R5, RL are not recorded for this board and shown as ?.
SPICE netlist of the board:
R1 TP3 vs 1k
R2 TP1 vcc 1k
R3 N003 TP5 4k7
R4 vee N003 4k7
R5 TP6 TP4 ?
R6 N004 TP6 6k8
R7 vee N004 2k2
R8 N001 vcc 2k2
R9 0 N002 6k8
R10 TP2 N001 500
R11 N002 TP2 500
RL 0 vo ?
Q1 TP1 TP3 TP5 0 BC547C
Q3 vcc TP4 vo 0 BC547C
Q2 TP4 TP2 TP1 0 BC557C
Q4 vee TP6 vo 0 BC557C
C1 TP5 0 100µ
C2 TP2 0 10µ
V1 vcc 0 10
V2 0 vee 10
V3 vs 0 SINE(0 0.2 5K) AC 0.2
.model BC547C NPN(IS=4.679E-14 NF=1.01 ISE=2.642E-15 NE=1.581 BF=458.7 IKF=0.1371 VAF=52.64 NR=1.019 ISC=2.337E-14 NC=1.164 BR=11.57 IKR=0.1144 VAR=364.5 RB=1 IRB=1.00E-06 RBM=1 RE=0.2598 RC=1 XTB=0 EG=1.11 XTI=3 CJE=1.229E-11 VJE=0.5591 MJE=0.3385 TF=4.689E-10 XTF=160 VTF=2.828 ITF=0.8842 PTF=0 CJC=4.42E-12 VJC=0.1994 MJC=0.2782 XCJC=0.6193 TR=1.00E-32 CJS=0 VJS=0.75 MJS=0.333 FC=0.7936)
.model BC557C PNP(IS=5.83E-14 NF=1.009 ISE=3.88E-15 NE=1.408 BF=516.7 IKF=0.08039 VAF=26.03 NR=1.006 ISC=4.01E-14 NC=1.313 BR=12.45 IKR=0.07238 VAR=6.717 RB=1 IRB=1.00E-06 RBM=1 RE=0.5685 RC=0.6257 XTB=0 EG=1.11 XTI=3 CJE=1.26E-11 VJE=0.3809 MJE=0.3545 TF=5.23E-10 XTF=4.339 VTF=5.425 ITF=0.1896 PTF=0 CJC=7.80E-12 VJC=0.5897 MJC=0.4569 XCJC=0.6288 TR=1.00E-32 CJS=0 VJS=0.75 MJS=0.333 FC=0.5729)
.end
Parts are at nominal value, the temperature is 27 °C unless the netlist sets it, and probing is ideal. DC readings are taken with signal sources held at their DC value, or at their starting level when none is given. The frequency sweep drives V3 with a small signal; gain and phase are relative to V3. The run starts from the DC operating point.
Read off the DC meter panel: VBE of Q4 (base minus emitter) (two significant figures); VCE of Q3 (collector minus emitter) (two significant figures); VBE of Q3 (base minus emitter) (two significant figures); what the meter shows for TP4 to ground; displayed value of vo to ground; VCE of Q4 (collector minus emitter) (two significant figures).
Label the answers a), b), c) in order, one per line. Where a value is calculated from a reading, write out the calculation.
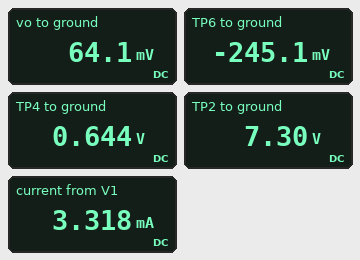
a) -245.1 mV - 64.1 mV = -310 mV
b) 10 V - 64.1 mV = 9.9 V
c) 644 mV - 64.1 mV = 580 mV
d) 0.644 V
e) 64.1 mV
f) -10 V - 64.1 mV = -10 V
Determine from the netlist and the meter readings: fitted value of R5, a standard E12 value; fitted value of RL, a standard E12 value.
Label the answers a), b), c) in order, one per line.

a) 820 Ω
b) 270 Ω
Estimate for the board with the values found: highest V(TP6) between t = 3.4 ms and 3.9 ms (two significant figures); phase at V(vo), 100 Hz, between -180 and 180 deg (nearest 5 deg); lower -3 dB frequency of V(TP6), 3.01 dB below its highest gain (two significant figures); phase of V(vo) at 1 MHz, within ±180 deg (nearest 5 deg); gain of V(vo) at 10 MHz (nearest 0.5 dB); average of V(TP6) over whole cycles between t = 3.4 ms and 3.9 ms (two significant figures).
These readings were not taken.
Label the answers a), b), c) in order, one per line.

a) 6.5 V
b) -150 deg
c) 56 Hz
d) 115 deg
e) 17.5 dB
f) 920 mV
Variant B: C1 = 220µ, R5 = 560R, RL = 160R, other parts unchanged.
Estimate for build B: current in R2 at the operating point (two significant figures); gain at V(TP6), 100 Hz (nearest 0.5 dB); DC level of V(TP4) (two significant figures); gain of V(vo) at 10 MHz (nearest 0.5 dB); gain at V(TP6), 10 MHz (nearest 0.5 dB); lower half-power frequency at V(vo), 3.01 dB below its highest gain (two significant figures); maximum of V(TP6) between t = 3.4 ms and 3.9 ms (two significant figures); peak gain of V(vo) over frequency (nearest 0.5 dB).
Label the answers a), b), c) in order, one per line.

a) 2.1 mA
b) 49.5 dB
c) 370 mV
d) 3.0 dB
e) 11.0 dB
f) 340 kHz
g) 6.9 V
h) 12.5 dB
